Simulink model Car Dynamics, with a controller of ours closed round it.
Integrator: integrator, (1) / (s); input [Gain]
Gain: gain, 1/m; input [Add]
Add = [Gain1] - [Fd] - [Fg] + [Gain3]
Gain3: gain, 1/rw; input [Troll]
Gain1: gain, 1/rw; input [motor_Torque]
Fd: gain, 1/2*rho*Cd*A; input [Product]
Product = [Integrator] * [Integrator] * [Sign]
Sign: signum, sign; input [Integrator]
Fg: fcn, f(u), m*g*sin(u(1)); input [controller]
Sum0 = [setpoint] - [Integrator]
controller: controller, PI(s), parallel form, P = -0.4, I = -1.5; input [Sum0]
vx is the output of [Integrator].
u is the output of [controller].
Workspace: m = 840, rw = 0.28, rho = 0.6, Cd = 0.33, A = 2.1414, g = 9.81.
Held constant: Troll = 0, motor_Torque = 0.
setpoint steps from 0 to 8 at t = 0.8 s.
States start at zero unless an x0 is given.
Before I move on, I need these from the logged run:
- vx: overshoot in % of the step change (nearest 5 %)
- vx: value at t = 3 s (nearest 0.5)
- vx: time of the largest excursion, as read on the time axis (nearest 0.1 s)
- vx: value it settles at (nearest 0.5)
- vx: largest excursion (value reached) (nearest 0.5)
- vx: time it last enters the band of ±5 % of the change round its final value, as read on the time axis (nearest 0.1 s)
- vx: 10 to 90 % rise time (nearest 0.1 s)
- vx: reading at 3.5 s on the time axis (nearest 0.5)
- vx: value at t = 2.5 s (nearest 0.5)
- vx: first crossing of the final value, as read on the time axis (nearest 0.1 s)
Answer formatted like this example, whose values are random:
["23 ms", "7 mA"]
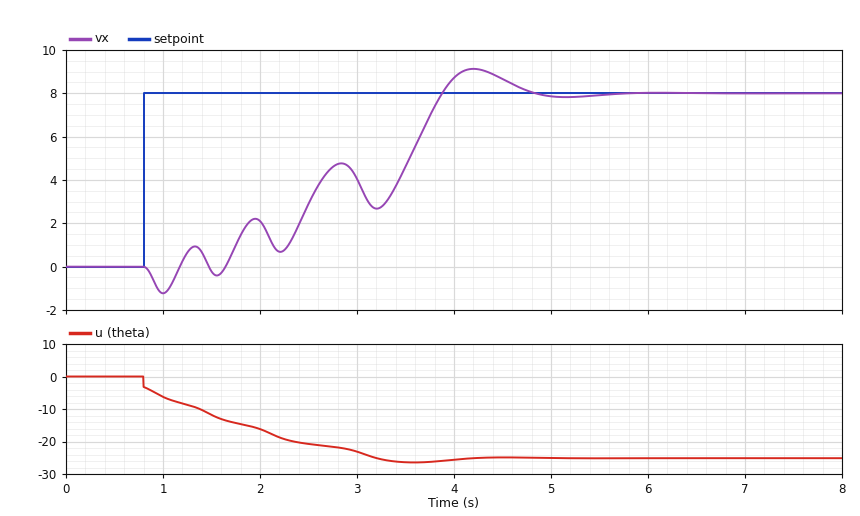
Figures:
["15 %", "4.0", "4.2 s", "8.0", "9.0", "4.6 s", "2.5 s", "4.5", "3.0", "3.9 s"]
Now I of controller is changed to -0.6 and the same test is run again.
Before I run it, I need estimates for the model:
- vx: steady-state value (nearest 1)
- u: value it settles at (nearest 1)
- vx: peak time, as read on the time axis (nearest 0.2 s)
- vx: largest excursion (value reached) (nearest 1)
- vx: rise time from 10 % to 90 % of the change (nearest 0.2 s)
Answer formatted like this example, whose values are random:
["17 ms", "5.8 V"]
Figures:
["8", "-6", "3.2 s", "8", "0.8 s"]
